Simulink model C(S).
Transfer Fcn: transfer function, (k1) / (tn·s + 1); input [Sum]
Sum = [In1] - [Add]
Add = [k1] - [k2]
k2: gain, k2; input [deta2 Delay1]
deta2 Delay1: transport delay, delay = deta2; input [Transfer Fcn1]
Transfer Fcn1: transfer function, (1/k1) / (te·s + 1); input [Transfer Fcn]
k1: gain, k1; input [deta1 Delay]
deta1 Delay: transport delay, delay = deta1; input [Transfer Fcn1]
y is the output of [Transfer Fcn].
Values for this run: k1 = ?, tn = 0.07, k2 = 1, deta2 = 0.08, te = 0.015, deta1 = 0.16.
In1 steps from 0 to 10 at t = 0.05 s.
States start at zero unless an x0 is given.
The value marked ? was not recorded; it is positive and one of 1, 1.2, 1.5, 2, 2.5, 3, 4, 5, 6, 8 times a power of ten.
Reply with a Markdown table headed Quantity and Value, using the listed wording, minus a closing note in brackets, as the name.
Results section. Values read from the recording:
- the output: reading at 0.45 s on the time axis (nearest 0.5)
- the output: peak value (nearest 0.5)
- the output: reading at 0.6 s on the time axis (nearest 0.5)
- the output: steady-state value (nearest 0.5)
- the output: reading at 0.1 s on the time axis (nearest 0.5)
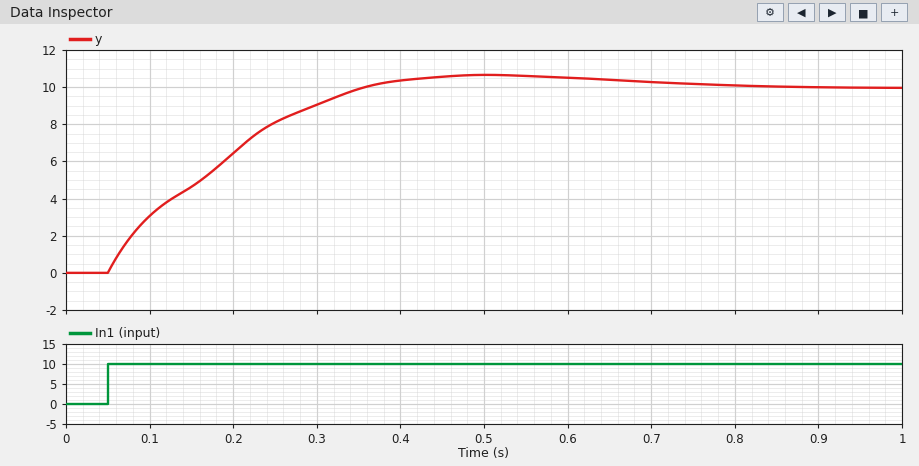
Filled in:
| Quantity | Value |
|---|---|
| the output: reading at 0.45 s on the time axis | 10.5 |
| the output: peak value | 10.5 |
| the output: reading at 0.6 s on the time axis | 10.5 |
| the output: steady-state value | 10.0 |
| the output: reading at 0.1 s on the time axis | 3.0 |
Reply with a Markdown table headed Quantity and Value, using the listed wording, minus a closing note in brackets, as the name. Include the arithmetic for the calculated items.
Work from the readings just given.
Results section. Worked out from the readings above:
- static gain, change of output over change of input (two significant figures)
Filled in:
| Quantity | Value |
|---|---|
| static gain, change of output over change of input | (10 - 0) / (10 - 0) = 1.0 |
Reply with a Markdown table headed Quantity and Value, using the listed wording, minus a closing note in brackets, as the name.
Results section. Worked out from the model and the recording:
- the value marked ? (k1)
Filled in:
| Quantity | Value |
|---|---|
| the value marked ? | 0.6 |
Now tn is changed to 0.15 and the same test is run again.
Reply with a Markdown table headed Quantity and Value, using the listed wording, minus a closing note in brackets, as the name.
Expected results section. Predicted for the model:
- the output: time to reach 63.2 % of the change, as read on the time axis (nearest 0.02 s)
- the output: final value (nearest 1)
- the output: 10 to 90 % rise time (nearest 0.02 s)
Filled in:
| Quantity | Value |
|---|---|
| the output: time to reach 63.2 % of the change, as read on the time axis | 0.30 s |
| the output: final value | 10 |
| the output: 10 to 90 % rise time | 0.48 s |
